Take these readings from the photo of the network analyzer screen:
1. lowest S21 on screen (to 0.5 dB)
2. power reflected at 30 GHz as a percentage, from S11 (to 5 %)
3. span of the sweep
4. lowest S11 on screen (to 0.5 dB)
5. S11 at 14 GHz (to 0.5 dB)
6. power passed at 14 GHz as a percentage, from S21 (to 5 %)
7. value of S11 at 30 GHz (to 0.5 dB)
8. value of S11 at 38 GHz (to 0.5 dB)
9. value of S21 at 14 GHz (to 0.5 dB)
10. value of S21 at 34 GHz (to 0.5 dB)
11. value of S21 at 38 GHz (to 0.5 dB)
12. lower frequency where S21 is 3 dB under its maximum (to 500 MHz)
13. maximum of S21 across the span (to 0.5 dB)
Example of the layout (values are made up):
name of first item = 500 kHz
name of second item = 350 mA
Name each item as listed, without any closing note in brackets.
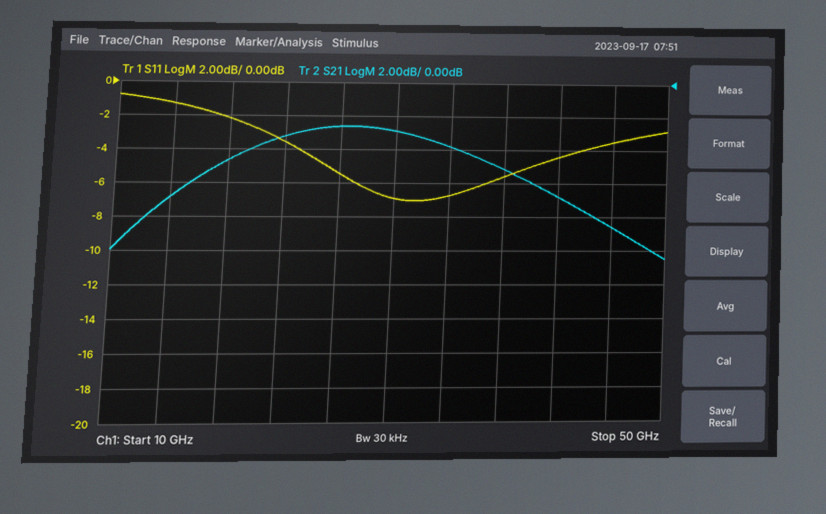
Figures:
lowest S21 on screen = -10.5 dB
power reflected at 30 GHz as a percentage, from S11 = 20 %
span of the sweep = 40 GHz
lowest S11 on screen = -7.0 dB
S11 at 14 GHz = -1.5 dB
power passed at 14 GHz as a percentage, from S21 = 20 %
value of S11 at 30 GHz = -7.0 dB
value of S11 at 38 GHz = -5.5 dB
value of S21 at 14 GHz = -7.0 dB
value of S21 at 34 GHz = -4.0 dB
value of S21 at 38 GHz = -5.0 dB
lower frequency where S21 is 3 dB under its maximum = 16.0 GHz
maximum of S21 across the span = -2.5 dB
